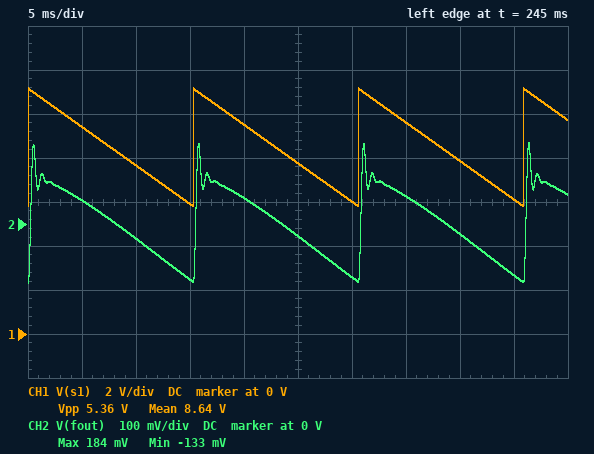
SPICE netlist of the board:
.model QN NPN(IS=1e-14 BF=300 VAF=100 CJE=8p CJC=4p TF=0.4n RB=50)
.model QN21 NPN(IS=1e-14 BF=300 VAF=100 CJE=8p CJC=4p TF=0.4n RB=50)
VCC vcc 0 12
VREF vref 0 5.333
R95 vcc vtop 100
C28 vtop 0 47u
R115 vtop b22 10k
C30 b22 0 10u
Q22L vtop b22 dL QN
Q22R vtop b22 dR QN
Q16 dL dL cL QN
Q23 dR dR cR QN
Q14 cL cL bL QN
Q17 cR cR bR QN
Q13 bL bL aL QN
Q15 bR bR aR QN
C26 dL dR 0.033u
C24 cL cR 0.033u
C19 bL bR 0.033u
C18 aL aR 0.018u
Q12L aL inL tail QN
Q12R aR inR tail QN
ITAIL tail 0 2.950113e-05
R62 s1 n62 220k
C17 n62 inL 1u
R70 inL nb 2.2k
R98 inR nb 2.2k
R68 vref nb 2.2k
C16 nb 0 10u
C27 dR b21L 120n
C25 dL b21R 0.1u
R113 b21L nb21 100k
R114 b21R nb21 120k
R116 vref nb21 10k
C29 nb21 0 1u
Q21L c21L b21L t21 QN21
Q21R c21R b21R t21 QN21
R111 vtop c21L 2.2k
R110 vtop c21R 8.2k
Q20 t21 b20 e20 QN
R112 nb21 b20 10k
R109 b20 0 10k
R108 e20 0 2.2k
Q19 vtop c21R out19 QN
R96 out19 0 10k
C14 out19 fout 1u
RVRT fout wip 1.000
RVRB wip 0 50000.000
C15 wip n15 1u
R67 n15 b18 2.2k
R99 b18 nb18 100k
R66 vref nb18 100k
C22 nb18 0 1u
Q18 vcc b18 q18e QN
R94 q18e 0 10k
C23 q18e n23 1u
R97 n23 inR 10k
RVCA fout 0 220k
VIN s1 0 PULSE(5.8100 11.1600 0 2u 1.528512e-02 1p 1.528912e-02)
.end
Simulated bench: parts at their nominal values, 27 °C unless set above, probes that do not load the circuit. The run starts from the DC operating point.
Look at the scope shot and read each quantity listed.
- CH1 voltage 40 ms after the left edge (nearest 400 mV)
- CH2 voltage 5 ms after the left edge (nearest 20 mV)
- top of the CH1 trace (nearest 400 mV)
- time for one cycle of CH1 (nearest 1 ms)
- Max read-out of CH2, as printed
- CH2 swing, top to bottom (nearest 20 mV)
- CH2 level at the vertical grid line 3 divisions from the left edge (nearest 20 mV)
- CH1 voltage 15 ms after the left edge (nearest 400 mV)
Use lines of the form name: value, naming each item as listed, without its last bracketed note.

CH1 voltage 40 ms after the left edge: 8.0 V
CH2 voltage 5 ms after the left edge: 60 mV
top of the CH1 trace: 11.2 V
time for one cycle of CH1: 15 ms
Max read-out of CH2, as printed: 184 mV
CH2 swing, top to bottom: 320 mV
CH2 level at the vertical grid line 3 divisions from the left edge: -120 mV
CH1 voltage 15 ms after the left edge: 6.0 V
